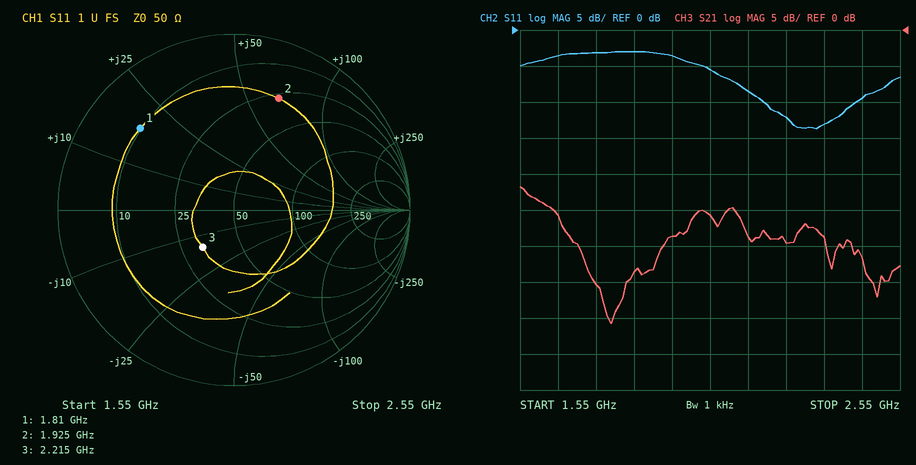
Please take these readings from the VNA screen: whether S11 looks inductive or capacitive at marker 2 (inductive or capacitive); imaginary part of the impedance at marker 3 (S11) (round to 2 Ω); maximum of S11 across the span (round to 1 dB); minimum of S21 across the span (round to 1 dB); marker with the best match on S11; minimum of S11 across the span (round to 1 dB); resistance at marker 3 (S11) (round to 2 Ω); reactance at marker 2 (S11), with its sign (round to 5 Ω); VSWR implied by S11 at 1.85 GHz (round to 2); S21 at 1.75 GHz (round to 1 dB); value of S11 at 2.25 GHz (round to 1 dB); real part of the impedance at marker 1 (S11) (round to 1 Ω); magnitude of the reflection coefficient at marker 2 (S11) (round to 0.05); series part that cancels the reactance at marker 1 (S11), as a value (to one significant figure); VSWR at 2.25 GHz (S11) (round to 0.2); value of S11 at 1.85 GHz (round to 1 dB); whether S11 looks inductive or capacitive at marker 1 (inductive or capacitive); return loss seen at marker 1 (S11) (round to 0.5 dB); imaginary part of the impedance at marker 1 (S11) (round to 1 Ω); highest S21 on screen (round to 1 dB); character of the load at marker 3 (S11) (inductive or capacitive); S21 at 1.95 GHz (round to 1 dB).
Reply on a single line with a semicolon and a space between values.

inductive; -14 Ω; -3 dB; -41 dB; marker 3; -14 dB; 32 Ω; +65 Ω; 6; -35 dB; -12 dB; 10 Ω; 0.70; 5 pF; 1.6; -3 dB; inductive; 3.0 dB; +18 Ω; -22 dB; capacitive; -29 dB
